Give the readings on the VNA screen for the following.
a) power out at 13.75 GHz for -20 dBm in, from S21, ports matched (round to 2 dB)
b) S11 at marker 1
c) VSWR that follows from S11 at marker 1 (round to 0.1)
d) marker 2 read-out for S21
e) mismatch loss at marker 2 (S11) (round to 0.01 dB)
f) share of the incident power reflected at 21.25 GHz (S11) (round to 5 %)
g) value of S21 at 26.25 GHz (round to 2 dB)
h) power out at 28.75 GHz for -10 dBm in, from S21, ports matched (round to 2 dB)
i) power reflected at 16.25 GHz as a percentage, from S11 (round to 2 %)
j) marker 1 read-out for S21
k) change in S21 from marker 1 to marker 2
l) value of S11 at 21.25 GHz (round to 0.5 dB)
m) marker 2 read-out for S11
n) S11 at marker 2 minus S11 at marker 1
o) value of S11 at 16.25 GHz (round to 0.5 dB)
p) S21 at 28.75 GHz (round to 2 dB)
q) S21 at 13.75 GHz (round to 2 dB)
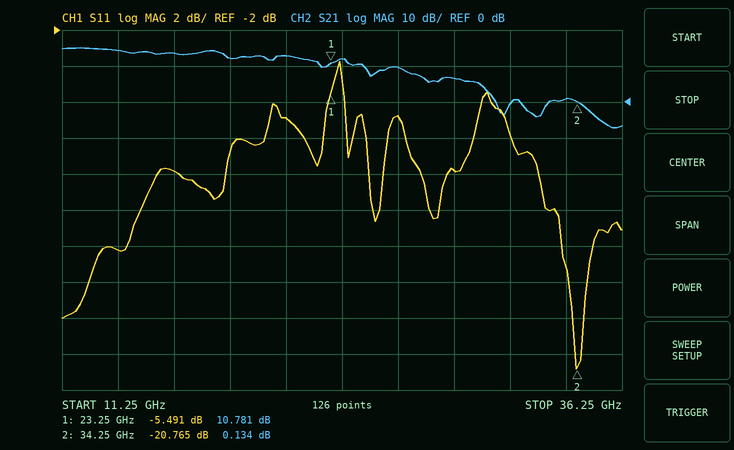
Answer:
-6 dBm
-5.491 dB
3.3
0.134 dB
0.04 dB
20 %
10 dB
-4 dBm
10 %
10.781 dB
-10.647 dB
-7.0 dB
-20.765 dB
-15.274 dB
-10.0 dB
6 dB
14 dB
